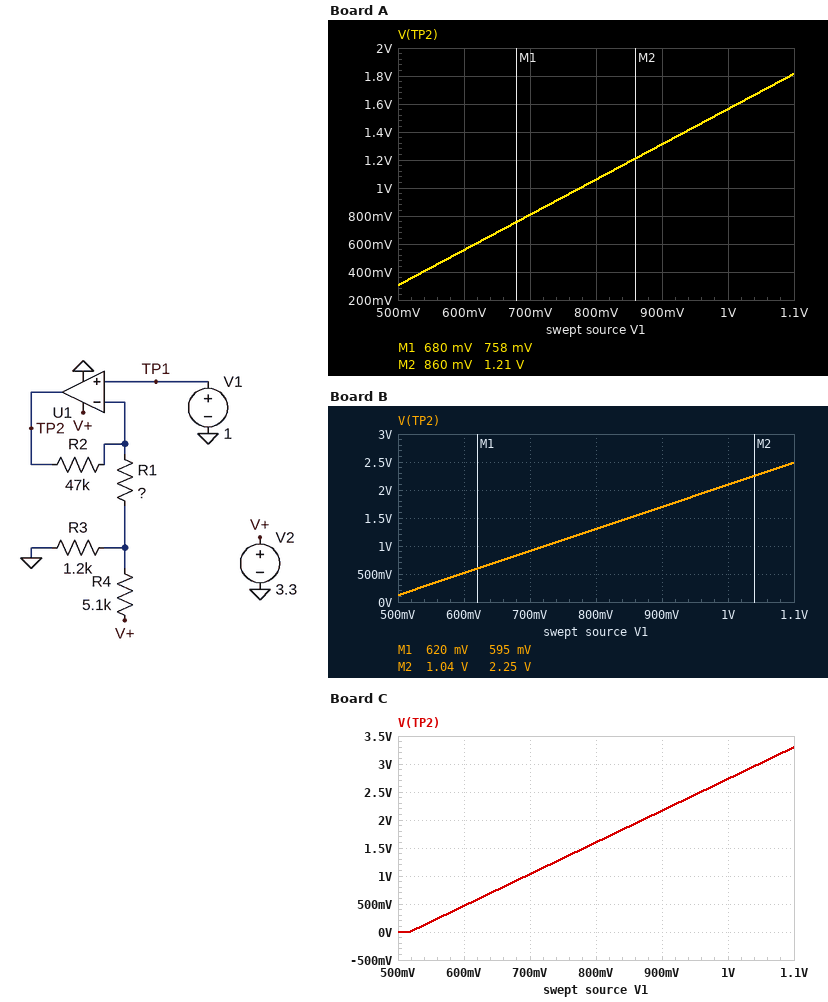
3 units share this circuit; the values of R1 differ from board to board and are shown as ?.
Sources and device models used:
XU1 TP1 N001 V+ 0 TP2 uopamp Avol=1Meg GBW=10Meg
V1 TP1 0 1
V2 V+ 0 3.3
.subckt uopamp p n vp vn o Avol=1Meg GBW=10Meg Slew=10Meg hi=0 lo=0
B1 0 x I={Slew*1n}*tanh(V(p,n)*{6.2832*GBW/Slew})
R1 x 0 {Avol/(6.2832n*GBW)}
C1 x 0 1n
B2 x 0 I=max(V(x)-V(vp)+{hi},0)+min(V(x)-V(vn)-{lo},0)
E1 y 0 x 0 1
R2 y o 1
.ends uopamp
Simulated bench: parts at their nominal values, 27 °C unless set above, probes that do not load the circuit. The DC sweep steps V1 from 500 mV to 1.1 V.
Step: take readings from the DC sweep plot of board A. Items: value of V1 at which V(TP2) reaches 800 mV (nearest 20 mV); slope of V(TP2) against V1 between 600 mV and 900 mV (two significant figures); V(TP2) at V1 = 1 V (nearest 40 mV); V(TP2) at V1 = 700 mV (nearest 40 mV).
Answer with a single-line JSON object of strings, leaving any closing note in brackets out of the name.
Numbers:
{"value of V1 at which V(TP2) reaches 800 mV": "700 mV", "slope of V(TP2) against V1 between 600 mV and 900 mV": "2.5 V/V", "V(TP2) at V1 = 1 V": "1.56 V", "V(TP2) at V1 = 700 mV": "800 mV"}
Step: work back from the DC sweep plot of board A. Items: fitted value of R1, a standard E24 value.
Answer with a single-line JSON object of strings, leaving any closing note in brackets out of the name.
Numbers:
{"fitted value of R1, a standard E24 value": "30 kΩ"}
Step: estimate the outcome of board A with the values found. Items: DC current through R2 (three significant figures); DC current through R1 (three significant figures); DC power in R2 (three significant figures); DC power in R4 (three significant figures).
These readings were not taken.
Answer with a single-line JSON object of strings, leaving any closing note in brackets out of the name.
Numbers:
{"DC current through R2": "12.0 µA", "DC current through R1": "12.0 µA", "DC power in R2": "6.76 µW", "DC power in R4": "1.39 mW"}
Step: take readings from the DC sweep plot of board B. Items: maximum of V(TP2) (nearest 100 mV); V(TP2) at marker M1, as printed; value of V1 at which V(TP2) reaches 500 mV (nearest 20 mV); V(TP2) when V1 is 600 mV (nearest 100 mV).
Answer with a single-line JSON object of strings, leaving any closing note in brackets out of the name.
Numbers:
{"maximum of V(TP2)": "2.5 V", "V(TP2) at marker M1, as printed": "595 mV", "value of V1 at which V(TP2) reaches 500 mV": "600 mV", "V(TP2) when V1 is 600 mV": "500 mV"}
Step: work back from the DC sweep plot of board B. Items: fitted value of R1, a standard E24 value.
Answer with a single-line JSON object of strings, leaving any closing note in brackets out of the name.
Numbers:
{"fitted value of R1, a standard E24 value": "15 kΩ"}
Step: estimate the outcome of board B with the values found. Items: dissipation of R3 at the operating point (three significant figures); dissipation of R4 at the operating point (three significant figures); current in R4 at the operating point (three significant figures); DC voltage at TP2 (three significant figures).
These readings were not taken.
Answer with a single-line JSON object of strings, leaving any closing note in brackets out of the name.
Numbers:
{"dissipation of R3 at the operating point": "353 µW", "dissipation of R4 at the operating point": "1.38 mW", "current in R4 at the operating point": "519 µA", "DC voltage at TP2": "2.09 V"}
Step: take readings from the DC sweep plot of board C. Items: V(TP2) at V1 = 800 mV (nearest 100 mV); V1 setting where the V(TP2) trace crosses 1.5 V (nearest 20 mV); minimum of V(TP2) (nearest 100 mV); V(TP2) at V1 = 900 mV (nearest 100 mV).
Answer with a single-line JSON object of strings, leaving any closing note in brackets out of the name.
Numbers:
{"V(TP2) at V1 = 800 mV": "1.6 V", "V1 setting where the V(TP2) trace crosses 1.5 V": "780 mV", "minimum of V(TP2)": "0 V", "V(TP2) at V1 = 900 mV": "2.2 V"}
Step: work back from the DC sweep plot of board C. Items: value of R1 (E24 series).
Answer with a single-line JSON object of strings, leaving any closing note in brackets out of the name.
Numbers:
{"value of R1": "9.1 kΩ"}
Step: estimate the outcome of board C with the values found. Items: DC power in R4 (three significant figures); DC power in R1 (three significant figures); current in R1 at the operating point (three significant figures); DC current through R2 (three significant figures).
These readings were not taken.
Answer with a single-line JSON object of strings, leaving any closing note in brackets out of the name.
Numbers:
{"DC power in R4": "1.36 mW", "DC power in R1": "12.4 µW", "current in R1 at the operating point": "36.9 µA", "DC current through R2": "36.9 µA"}
